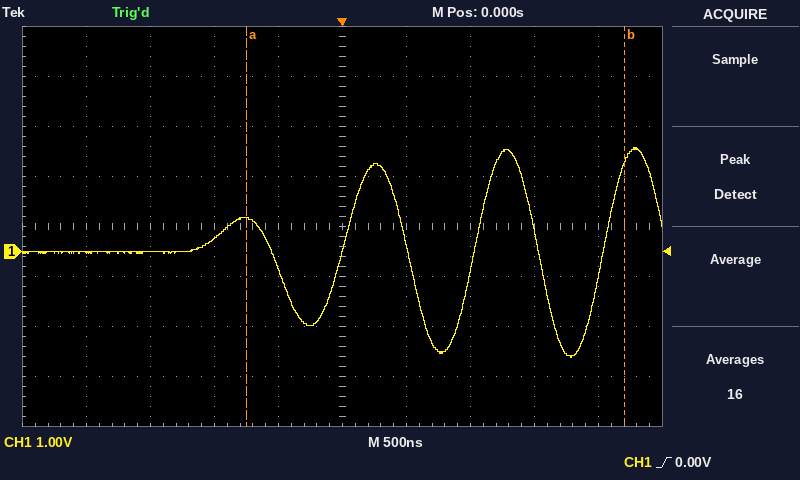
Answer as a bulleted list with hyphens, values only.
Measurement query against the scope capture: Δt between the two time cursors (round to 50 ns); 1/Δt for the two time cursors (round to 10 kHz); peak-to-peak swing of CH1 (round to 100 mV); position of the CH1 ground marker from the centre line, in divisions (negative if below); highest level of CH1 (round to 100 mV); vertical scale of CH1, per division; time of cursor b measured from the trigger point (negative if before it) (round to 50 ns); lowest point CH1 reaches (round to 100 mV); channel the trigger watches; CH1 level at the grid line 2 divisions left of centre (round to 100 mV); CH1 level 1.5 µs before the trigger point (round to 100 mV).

- 2.95 µs
- 340 kHz
- 4.2 V
- -0.5 div
- 2.1 V
- 1 V
- +2.20 µs
- -2.1 V
- CH1
- 300 mV
- 0.0 V
